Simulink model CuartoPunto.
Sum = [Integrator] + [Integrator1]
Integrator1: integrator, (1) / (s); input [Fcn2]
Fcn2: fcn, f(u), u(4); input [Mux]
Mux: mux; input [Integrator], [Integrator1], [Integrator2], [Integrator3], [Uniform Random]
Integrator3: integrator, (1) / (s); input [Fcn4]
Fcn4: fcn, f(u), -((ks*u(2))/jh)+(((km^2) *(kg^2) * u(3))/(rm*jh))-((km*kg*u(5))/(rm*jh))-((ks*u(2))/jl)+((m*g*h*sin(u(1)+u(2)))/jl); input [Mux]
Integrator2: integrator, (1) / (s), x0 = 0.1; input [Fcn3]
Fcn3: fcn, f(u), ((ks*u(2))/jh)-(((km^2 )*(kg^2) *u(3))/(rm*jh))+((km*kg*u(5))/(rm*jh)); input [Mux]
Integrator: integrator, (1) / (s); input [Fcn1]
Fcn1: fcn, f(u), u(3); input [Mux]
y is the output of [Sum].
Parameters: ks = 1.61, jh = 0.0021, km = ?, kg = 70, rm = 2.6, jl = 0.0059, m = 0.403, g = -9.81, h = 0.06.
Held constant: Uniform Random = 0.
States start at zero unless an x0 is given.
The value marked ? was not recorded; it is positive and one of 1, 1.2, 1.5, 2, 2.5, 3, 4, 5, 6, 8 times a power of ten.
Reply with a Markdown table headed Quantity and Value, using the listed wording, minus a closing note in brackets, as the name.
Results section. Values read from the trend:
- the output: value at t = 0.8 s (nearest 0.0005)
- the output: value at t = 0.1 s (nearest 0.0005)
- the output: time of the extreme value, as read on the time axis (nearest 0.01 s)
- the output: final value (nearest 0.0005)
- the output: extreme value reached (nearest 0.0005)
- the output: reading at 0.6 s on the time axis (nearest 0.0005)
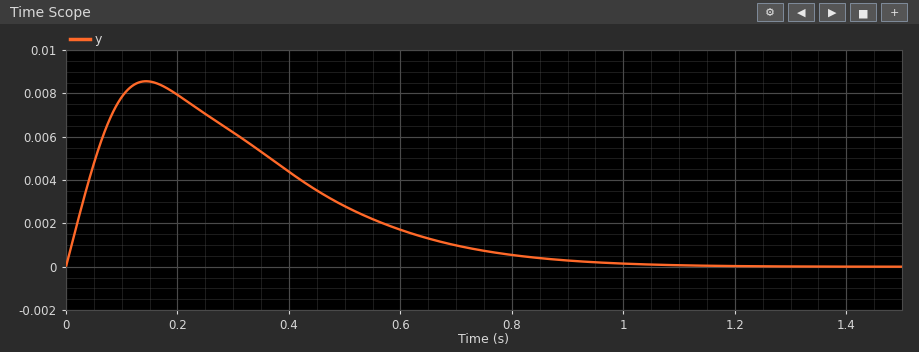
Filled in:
| Quantity | Value |
|---|---|
| the output: value at t = 0.8 s | 0.0005 |
| the output: value at t = 0.1 s | 0.0080 |
| the output: time of the extreme value, as read on the time axis | 0.14 s |
| the output: final value | 0.0000 |
| the output: extreme value reached | 0.0085 |
| the output: reading at 0.6 s on the time axis | 0.0015 |
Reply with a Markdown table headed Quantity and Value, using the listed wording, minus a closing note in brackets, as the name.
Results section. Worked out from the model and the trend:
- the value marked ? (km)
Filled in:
| Quantity | Value |
|---|---|
| the value marked ? | 0.006 |
